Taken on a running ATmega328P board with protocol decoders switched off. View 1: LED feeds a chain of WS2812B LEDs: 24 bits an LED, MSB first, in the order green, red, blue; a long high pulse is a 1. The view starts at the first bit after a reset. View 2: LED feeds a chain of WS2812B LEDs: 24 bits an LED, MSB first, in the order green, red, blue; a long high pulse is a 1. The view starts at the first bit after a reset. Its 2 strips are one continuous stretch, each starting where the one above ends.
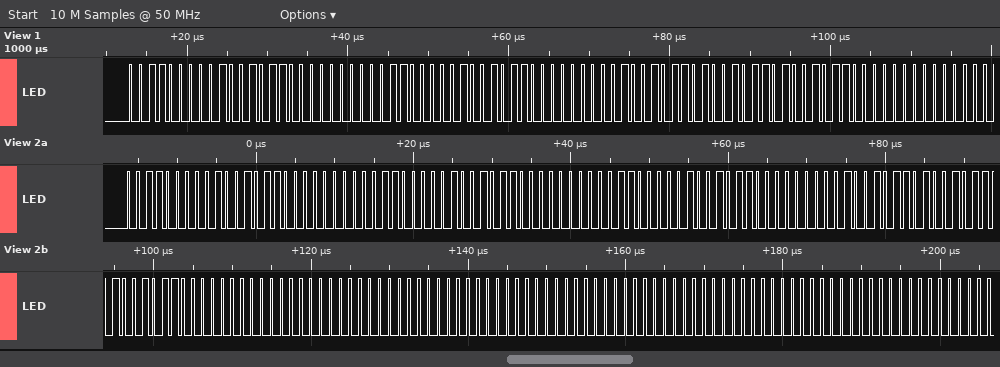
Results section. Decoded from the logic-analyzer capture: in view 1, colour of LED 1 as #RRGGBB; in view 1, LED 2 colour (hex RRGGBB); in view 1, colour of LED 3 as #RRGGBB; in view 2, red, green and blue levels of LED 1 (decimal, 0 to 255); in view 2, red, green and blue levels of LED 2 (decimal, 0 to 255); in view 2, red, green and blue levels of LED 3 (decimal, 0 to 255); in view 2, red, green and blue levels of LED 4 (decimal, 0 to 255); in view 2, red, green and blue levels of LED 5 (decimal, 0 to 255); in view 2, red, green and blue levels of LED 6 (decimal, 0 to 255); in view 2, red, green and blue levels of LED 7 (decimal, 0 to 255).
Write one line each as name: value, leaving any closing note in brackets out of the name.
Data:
in view 1, colour of LED 1 as #RRGGBB: #4B3000
in view 1, LED 2 colour: #4B3000
in view 1, colour of LED 3 as #RRGGBB: #4B4B4B
in view 2, red, green and blue levels of LED 1: 75, 48, 0
in view 2, red, green and blue levels of LED 2: 75, 48, 0
in view 2, red, green and blue levels of LED 3: 75, 48, 0
in view 2, red, green and blue levels of LED 4: 75, 75, 75
in view 2, red, green and blue levels of LED 5: 0, 0, 0
in view 2, red, green and blue levels of LED 6: 0, 0, 0
in view 2, red, green and blue levels of LED 7: 0, 0, 0
